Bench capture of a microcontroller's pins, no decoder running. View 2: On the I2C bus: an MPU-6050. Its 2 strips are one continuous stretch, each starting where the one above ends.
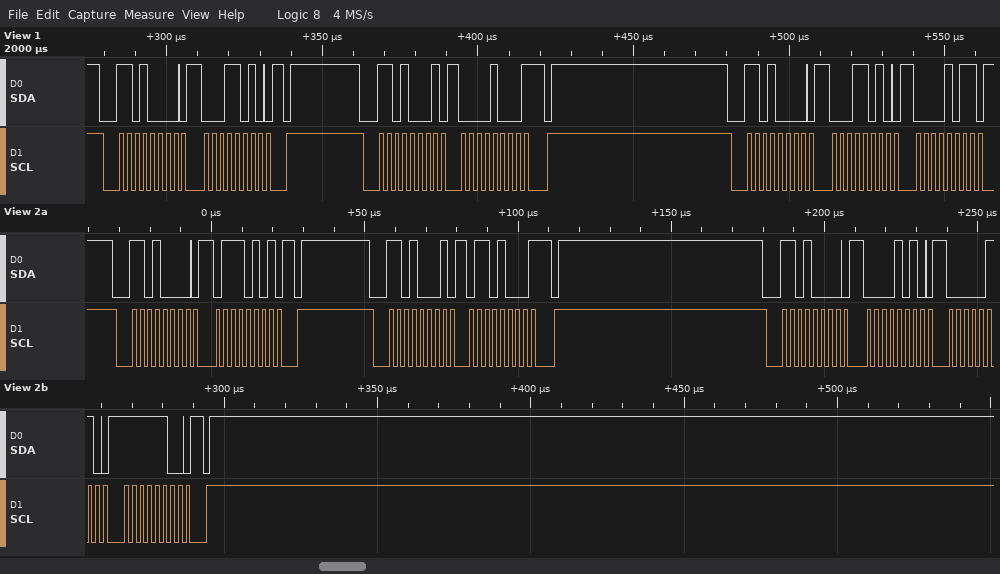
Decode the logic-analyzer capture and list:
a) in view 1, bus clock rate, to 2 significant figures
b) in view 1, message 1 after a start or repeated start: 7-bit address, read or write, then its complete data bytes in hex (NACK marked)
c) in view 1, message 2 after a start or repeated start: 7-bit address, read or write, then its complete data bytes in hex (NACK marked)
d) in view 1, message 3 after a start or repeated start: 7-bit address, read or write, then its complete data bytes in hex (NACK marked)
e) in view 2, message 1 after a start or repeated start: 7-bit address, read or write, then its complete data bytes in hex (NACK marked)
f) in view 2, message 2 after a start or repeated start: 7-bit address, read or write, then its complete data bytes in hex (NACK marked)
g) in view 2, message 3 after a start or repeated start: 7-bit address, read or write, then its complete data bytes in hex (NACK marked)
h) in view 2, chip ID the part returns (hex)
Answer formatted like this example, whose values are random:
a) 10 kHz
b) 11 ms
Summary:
a) 400 kHz
b) 0x68 write: 1A
c) 0x68 read: 08 NACK
d) 0x68 write: 1A 0B
e) 0x68 write: 75
f) 0x68 read: 68 NACK
g) 0x68 write: 0A 06 FC
h) 0x68
